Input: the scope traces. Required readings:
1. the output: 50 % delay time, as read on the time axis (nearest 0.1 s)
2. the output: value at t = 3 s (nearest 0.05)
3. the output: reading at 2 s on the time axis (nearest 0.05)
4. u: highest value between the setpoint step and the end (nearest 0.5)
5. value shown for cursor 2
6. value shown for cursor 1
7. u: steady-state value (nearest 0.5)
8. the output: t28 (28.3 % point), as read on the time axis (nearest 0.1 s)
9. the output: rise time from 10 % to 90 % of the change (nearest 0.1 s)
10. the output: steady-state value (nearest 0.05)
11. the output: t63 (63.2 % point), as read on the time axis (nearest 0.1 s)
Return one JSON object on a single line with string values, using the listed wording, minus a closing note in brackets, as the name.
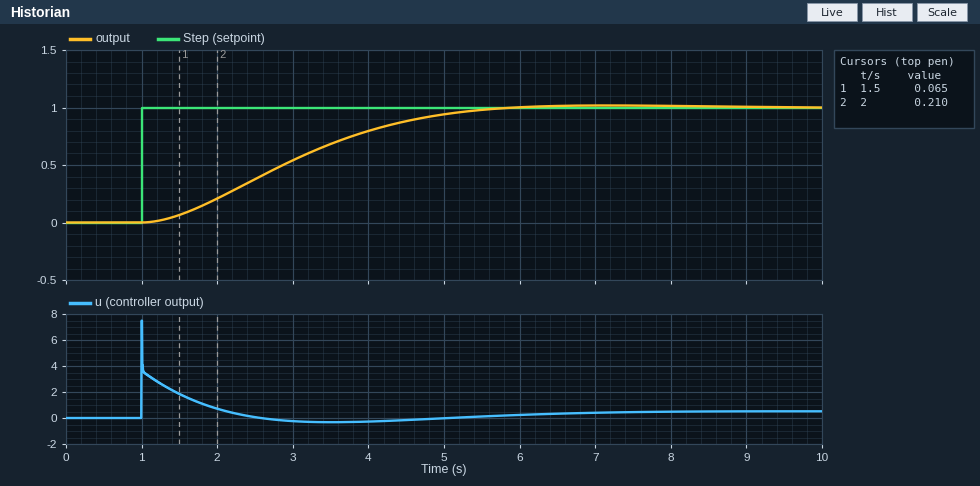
{"the output: 50 % delay time, as read on the time axis": "2.9 s", "the output: value at t = 3 s": "0.55", "the output: reading at 2 s on the time axis": "0.20", "u: highest value between the setpoint step and the end": "7.5", "value shown for cursor 2": "0.210", "value shown for cursor 1": "0.065", "u: steady-state value": "0.5", "the output: t28 (28.3 % point), as read on the time axis": "2.2 s", "the output: rise time from 10 % to 90 % of the change": "3.0 s", "the output: steady-state value": "1.00", "the output: t63 (63.2 % point), as read on the time axis": "3.3 s"}
